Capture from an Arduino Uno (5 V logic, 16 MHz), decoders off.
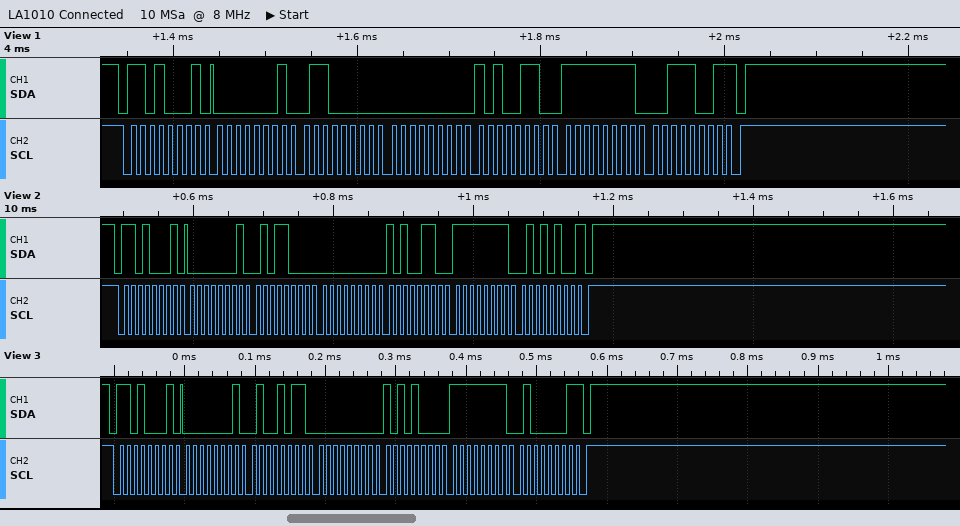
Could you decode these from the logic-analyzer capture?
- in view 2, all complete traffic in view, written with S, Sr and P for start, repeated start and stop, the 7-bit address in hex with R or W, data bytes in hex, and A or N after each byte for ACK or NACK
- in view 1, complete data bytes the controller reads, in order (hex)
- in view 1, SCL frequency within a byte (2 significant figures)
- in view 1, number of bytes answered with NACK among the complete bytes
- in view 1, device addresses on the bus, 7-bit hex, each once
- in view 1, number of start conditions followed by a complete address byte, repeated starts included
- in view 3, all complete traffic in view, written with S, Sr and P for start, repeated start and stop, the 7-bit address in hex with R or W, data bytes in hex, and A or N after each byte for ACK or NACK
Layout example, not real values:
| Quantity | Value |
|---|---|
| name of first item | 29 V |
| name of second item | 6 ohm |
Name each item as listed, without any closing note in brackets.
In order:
| Quantity | Value |
|---|---|
| in view 2, all complete traffic in view, written with S, Sr and P for start, repeated start and stop, the 7-bit address in hex with R or W, data bytes in hex, and A or N after each byte for ACK or NACK | S 68R A 01 A 58 A 00 A A6 A FF A 54 N P |
| in view 1, complete data bytes the controller reads, in order | 01 60 00 A6 FF 39 |
| in view 1, SCL frequency within a byte | 100 kHz |
| in view 1, number of bytes answered with NACK among the complete bytes | 1 |
| in view 1, device addresses on the bus, 7-bit hex, each once | 0x68 |
| in view 1, number of start conditions followed by a complete address byte, repeated starts included | 1 |
| in view 3, all complete traffic in view, written with S, Sr and P for start, repeated start and stop, the 7-bit address in hex with R or W, data bytes in hex, and A or N after each byte for ACK or NACK | S 68R A 01 A 4B A 00 A A8 A FF A 41 N P |
